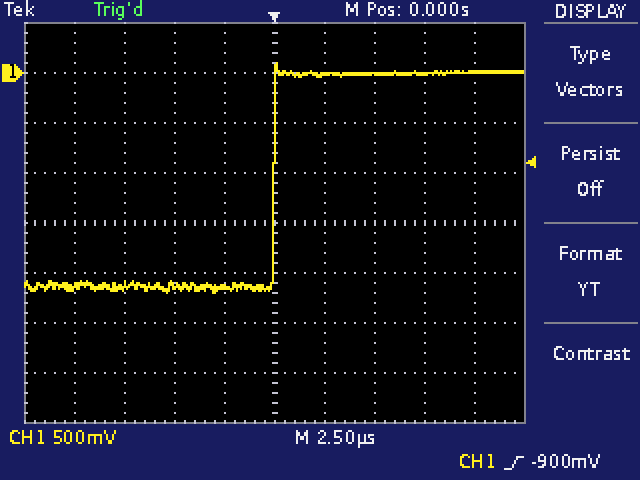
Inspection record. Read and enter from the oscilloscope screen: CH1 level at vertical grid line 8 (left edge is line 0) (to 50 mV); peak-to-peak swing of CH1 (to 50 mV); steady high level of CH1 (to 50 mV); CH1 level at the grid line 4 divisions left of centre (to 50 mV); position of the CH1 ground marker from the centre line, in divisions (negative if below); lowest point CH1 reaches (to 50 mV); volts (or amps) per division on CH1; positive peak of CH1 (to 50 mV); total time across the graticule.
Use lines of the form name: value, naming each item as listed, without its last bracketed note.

CH1 level at vertical grid line 8 (left edge is line 0): 0 mV
peak-to-peak swing of CH1: 2.30 V
steady high level of CH1: 0 mV
CH1 level at the grid line 4 divisions left of centre: -2.15 V
position of the CH1 ground marker from the centre line, in divisions: +3.0 div
lowest point CH1 reaches: -2.20 V
volts (or amps) per division on CH1: 500 mV
positive peak of CH1: 100 mV
total time across the graticule: 25 µs
